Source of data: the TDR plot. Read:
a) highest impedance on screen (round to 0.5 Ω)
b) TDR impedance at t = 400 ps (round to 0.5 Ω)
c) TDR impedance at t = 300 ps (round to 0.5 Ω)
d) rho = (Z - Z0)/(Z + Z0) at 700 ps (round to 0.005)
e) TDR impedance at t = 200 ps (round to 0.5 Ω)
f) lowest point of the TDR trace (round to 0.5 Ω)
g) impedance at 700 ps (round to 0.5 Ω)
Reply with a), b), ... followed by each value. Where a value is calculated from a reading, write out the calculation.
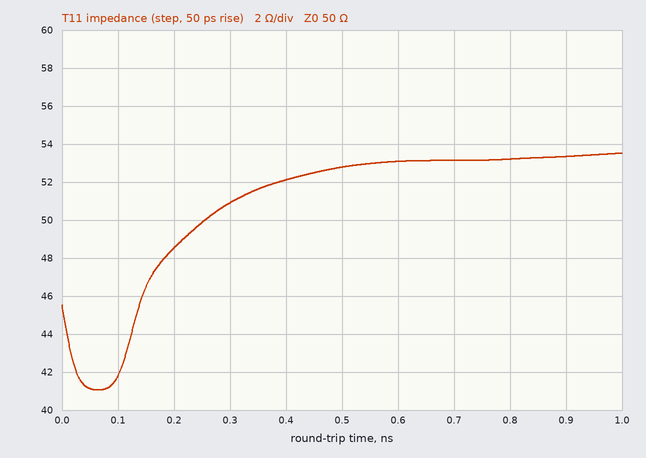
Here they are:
a) 53.5 Ω
b) 52.0 Ω
c) 51.0 Ω
d) (53 − 50)/(53 + 50) ≈ +0.0291, so +0.030 to the nearest 0.005
e) 48.5 Ω
f) 41.0 Ω
g) 53.0 Ω
